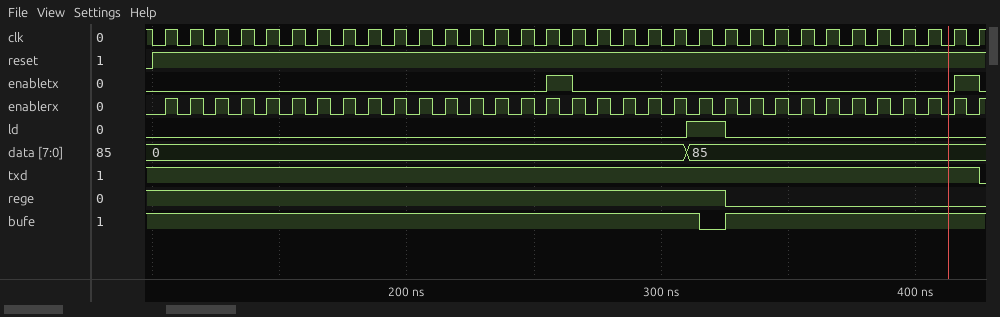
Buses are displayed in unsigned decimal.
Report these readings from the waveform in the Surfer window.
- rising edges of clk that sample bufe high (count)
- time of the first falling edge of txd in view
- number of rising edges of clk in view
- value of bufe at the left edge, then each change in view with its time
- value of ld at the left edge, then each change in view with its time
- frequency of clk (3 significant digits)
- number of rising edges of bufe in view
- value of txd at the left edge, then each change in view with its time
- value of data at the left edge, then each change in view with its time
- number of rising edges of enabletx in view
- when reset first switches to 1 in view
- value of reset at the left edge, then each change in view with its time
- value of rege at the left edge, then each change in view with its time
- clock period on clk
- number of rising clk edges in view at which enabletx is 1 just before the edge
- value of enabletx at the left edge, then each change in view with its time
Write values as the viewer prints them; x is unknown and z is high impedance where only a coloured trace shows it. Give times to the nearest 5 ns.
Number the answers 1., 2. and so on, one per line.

1. 32
2. 425 ns
3. 33
4. 1, 0 at 315 ns, 1 at 325 ns
5. 0, 1 at 310 ns, 0 at 325 ns
6. 100 MHz
7. 1
8. 1, 0 at 425 ns
9. 0, 85 at 310 ns
10. 2
11. 100 ns
12. 0, 1 at 100 ns
13. 1, 0 at 325 ns
14. 10 ns
15. 2
16. 0, 1 at 255 ns, 0 at 265 ns, 1 at 415 ns, 0 at 425 ns
